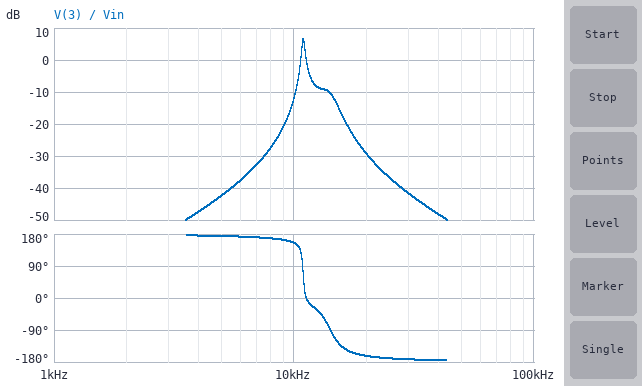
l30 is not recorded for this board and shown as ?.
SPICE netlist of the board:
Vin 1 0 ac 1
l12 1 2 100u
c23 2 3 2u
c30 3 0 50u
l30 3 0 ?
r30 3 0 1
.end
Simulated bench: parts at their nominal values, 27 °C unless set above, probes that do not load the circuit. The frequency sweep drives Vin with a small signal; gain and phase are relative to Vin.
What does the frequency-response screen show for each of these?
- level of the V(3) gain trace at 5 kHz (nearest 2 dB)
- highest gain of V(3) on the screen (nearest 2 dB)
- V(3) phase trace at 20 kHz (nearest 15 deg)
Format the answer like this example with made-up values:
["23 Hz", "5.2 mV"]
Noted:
["-42 dB", "6 dB", "-165 deg"]
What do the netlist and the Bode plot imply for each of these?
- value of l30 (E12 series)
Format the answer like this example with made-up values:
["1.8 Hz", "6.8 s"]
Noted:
["2.7 µH"]
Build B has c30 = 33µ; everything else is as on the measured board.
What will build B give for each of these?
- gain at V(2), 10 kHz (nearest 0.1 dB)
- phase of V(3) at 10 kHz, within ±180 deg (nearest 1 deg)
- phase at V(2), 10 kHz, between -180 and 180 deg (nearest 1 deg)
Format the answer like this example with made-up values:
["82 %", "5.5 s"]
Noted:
["14.6 dB", "163 deg", "-2 deg"]
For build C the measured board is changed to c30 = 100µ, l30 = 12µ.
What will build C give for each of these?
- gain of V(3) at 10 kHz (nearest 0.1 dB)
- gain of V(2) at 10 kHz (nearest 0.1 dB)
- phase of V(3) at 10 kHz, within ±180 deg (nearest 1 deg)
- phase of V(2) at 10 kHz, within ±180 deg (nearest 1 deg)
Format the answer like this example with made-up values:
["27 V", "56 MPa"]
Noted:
["-19.5 dB", "12.8 dB", "10 deg", "-1 deg"]
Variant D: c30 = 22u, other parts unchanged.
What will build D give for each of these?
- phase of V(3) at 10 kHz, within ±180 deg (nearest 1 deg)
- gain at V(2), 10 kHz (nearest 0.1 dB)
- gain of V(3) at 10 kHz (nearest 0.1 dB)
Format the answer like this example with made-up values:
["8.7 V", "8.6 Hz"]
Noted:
["166 deg", "14.5 dB", "-16.6 dB"]
